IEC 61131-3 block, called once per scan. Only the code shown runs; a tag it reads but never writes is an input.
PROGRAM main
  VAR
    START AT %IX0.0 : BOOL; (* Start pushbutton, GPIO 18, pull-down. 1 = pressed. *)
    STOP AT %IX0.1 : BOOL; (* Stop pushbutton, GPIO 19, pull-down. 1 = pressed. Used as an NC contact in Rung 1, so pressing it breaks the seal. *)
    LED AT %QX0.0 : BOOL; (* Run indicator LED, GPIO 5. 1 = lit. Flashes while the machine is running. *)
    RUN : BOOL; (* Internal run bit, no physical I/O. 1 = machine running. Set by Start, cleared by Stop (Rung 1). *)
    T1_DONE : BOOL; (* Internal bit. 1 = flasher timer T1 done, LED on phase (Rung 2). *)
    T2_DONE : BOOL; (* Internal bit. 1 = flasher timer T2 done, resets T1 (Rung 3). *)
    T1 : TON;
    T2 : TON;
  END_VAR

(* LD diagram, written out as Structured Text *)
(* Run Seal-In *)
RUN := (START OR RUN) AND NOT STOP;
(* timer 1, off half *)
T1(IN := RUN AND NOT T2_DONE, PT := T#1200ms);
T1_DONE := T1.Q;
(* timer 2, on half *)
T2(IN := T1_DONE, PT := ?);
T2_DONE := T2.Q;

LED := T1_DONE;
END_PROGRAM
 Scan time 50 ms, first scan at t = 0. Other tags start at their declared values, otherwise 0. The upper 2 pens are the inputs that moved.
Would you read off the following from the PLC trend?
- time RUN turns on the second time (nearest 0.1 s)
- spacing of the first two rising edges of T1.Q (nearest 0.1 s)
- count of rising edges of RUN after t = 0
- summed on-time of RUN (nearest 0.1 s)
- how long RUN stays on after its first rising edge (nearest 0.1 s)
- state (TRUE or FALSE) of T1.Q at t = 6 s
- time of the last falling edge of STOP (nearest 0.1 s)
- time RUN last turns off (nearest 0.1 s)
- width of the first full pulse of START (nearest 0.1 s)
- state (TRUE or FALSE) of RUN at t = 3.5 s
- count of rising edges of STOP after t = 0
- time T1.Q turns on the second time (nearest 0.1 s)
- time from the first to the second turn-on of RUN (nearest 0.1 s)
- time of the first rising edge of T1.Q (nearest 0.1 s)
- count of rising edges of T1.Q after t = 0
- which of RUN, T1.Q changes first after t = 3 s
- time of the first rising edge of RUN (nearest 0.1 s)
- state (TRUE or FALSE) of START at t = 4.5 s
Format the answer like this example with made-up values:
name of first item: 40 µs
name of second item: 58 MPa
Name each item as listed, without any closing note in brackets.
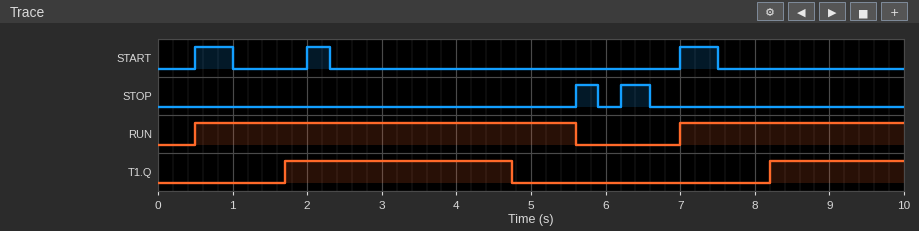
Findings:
time RUN turns on the second time: 7.0 s
spacing of the first two rising edges of T1.Q: 6.5 s
count of rising edges of RUN after t = 0: 2
summed on-time of RUN: 8.1 s
how long RUN stays on after its first rising edge: 5.1 s
state (TRUE or FALSE) of T1.Q at t = 6 s: FALSE
time of the last falling edge of STOP: 6.6 s
time RUN last turns off: 5.6 s
width of the first full pulse of START: 0.5 s
state (TRUE or FALSE) of RUN at t = 3.5 s: TRUE
count of rising edges of STOP after t = 0: 2
time T1.Q turns on the second time: 8.2 s
time from the first to the second turn-on of RUN: 6.5 s
time of the first rising edge of T1.Q: 1.7 s
count of rising edges of T1.Q after t = 0: 2
which of RUN, T1.Q changes first after t = 3 s: T1.Q
time of the first rising edge of RUN: 0.5 s
state (TRUE or FALSE) of START at t = 4.5 s: FALSE
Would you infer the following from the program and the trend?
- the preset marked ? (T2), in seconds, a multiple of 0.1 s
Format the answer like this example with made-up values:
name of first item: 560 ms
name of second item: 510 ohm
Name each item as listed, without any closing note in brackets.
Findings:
the preset marked ? (T2), in seconds, a multiple of 0.1 s: 3.0 s
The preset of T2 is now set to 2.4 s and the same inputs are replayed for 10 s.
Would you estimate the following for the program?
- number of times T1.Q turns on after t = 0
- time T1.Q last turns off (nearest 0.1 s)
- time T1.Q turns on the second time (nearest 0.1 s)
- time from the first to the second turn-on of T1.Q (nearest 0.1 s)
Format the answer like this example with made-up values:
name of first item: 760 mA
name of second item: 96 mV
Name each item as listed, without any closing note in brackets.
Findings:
number of times T1.Q turns on after t = 0: 3
time T1.Q last turns off: 5.6 s
time T1.Q turns on the second time: 5.4 s
time from the first to the second turn-on of T1.Q: 3.7 s
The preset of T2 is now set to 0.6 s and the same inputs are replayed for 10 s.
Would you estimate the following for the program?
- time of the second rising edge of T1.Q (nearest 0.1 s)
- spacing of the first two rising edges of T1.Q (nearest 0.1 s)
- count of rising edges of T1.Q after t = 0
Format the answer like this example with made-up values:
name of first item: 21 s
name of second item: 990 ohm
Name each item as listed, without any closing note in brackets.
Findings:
time of the second rising edge of T1.Q: 3.6 s
spacing of the first two rising edges of T1.Q: 1.9 s
count of rising edges of T1.Q after t = 0: 4
